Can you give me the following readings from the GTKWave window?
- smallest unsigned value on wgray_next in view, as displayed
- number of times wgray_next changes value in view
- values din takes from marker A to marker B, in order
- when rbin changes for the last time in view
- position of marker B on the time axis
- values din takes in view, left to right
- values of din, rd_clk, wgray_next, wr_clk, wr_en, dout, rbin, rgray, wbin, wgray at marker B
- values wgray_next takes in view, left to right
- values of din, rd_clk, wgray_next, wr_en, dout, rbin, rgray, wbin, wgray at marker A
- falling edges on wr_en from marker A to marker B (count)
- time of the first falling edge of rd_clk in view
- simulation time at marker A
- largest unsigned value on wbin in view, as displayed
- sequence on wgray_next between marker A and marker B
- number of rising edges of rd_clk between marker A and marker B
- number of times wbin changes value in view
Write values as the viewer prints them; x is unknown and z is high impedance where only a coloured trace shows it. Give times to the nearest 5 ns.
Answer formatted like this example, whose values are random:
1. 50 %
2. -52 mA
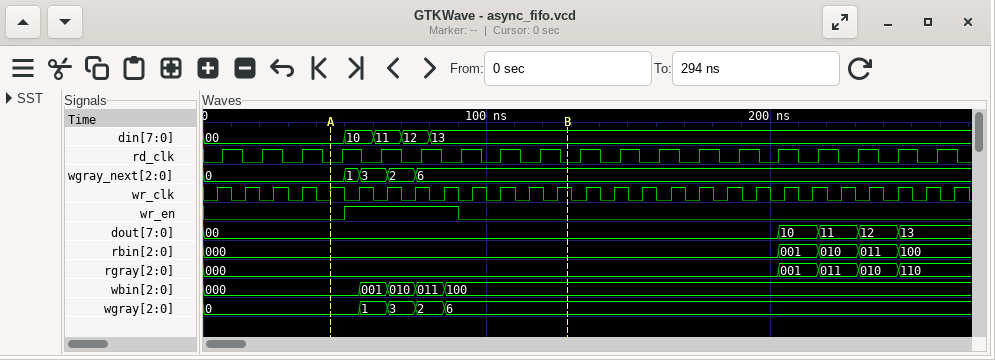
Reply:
1. 0
2. 4
3. 00, 10, 11, 12, 13
4. 245 ns
5. 130 ns
6. 00, 10, 11, 12, 13
7. din=13, rd_clk=0, wgray_next=6, wr_clk=1, wr_en=0, dout=00, rbin=000, rgray=000, wbin=100, wgray=6
8. 0, 1, 3, 2, 6
9. din=00, rd_clk=0, wgray_next=0, wr_en=0, dout=00, rbin=000, rgray=000, wbin=000, wgray=0
10. 1
11. 15 ns
12. 45 ns
13. 100
14. 0, 1, 3, 2, 6
15. 6
16. 4
